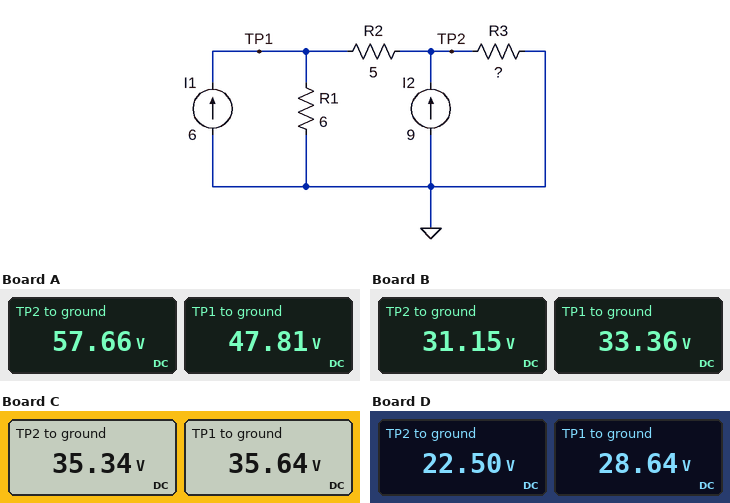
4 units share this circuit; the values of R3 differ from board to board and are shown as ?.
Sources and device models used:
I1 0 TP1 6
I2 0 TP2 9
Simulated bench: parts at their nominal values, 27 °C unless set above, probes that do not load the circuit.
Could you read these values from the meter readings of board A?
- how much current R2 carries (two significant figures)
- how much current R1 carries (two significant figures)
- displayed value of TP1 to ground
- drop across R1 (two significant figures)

2.0 A
8.0 A
47.81 V
48 V
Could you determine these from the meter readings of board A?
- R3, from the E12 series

8.2 Ω
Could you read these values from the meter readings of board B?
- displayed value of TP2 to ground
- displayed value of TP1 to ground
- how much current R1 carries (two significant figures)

31.15 V
33.36 V
5.6 A
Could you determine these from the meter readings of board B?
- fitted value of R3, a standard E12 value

3.3 Ω
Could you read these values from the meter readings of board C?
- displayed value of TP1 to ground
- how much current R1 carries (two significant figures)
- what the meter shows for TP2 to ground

35.64 V
5.9 A
35.34 V
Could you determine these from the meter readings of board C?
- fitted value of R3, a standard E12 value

3.9 Ω
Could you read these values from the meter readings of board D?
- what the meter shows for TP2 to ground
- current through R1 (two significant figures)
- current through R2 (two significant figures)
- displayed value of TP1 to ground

22.50 V
4.8 A
1.2 A
28.64 V
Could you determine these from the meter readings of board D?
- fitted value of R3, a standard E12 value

2.2 Ω
